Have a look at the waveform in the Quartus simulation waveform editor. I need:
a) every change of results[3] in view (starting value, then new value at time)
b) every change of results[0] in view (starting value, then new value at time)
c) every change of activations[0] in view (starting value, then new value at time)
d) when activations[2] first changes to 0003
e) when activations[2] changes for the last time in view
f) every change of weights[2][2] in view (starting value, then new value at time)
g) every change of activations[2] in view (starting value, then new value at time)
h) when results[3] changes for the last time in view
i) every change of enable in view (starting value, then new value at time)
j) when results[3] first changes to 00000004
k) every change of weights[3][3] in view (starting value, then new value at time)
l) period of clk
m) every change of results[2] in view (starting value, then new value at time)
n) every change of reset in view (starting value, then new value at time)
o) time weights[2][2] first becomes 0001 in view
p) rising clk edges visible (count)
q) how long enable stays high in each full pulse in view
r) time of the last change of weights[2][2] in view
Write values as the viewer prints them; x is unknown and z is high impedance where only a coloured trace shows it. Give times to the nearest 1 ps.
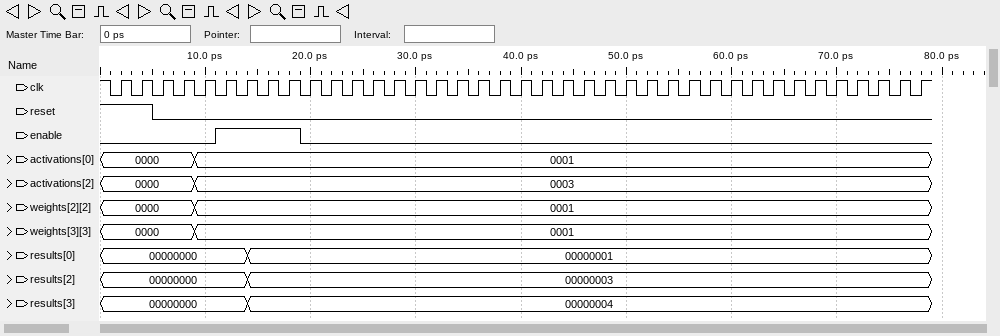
00000000, 00000004 at 14 ps
00000000, 00000001 at 14 ps
0000, 0001 at 9 ps
9 ps
9 ps
0000, 0001 at 9 ps
0000, 0003 at 9 ps
14 ps
0, 1 at 11 ps, 0 at 19 ps
14 ps
0000, 0001 at 9 ps
2 ps
00000000, 00000003 at 14 ps
1, 0 at 5 ps
9 ps
39
8 ps
9 ps
